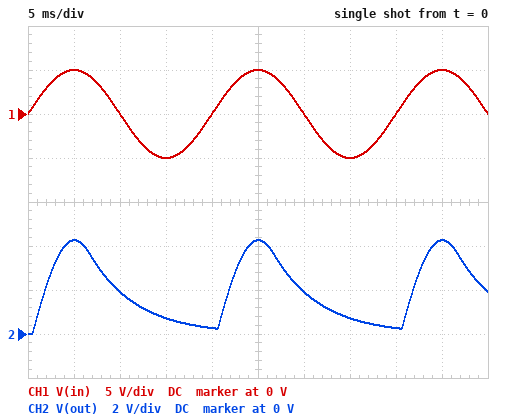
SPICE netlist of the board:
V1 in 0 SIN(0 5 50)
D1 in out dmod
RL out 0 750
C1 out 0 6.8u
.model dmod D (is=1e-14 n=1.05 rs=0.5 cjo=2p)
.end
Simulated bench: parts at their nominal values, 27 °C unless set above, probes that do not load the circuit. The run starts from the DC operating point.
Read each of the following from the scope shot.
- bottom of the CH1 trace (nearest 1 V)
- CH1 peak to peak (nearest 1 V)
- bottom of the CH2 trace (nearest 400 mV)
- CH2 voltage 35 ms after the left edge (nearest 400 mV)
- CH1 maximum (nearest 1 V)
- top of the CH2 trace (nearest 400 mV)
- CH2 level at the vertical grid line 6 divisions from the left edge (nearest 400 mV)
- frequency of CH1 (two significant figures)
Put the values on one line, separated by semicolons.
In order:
-5 V; 10 V; 0 V; 800 mV; 5 V; 4.4 V; 2.0 V; 50 Hz
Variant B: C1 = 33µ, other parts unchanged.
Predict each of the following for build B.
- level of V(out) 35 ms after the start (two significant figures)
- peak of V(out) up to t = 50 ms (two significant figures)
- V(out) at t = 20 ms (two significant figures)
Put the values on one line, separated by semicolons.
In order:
2.9 V; 4.3 V; 2.4 V
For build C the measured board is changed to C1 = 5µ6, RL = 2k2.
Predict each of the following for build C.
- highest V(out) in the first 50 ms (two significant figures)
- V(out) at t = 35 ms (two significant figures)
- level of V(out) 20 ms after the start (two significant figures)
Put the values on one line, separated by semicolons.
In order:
4.3 V; 2.0 V; 1.3 V
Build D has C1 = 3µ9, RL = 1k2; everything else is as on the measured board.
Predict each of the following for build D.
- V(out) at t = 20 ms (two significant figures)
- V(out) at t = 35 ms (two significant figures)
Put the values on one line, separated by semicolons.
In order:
210 mV; 620 mV
